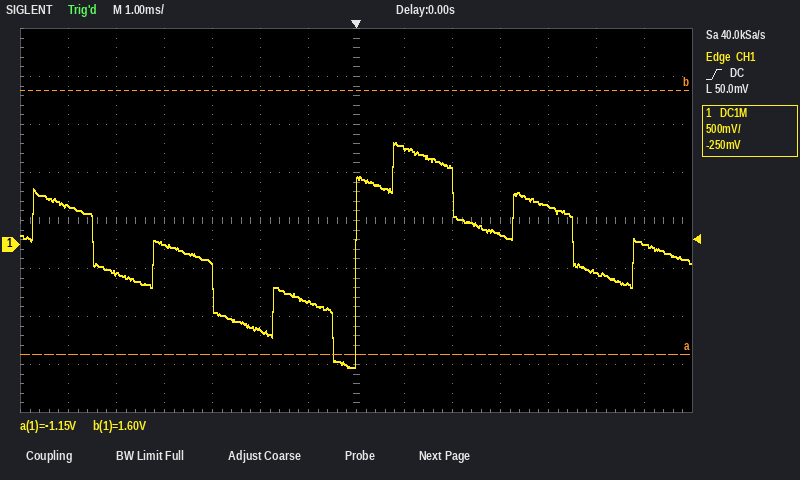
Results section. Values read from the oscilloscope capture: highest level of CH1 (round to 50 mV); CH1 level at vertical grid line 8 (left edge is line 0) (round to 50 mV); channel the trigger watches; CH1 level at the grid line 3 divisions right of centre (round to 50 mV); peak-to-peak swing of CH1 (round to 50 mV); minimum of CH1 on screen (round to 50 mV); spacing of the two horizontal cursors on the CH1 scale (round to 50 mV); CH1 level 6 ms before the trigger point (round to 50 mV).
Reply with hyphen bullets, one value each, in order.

- 1.05 V
- 1.00 V
- CH1
- 100 mV
- 2.35 V
- -1.30 V
- 2.75 V
- 400 mV
